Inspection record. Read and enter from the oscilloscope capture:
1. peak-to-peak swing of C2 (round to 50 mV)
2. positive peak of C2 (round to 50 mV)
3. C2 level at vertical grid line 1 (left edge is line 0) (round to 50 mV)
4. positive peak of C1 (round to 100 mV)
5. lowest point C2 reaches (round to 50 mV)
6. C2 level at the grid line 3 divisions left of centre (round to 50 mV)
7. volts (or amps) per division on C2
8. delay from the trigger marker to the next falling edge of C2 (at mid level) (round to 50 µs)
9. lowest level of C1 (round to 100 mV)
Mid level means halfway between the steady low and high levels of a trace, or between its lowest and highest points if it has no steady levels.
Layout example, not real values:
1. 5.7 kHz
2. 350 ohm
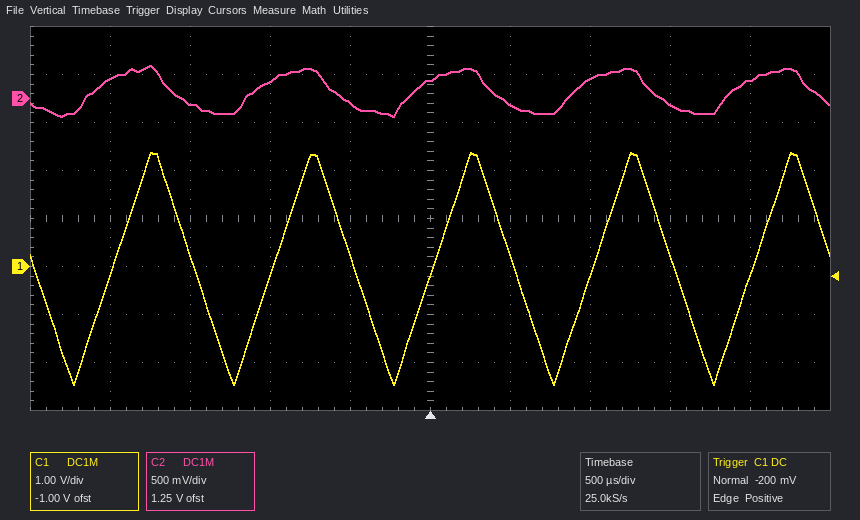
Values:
1. 550 mV
2. 350 mV
3. 200 mV
4. 2.4 V
5. -200 mV
6. -50 mV
7. 500 mV
8. 400 µs
9. -2.5 V
